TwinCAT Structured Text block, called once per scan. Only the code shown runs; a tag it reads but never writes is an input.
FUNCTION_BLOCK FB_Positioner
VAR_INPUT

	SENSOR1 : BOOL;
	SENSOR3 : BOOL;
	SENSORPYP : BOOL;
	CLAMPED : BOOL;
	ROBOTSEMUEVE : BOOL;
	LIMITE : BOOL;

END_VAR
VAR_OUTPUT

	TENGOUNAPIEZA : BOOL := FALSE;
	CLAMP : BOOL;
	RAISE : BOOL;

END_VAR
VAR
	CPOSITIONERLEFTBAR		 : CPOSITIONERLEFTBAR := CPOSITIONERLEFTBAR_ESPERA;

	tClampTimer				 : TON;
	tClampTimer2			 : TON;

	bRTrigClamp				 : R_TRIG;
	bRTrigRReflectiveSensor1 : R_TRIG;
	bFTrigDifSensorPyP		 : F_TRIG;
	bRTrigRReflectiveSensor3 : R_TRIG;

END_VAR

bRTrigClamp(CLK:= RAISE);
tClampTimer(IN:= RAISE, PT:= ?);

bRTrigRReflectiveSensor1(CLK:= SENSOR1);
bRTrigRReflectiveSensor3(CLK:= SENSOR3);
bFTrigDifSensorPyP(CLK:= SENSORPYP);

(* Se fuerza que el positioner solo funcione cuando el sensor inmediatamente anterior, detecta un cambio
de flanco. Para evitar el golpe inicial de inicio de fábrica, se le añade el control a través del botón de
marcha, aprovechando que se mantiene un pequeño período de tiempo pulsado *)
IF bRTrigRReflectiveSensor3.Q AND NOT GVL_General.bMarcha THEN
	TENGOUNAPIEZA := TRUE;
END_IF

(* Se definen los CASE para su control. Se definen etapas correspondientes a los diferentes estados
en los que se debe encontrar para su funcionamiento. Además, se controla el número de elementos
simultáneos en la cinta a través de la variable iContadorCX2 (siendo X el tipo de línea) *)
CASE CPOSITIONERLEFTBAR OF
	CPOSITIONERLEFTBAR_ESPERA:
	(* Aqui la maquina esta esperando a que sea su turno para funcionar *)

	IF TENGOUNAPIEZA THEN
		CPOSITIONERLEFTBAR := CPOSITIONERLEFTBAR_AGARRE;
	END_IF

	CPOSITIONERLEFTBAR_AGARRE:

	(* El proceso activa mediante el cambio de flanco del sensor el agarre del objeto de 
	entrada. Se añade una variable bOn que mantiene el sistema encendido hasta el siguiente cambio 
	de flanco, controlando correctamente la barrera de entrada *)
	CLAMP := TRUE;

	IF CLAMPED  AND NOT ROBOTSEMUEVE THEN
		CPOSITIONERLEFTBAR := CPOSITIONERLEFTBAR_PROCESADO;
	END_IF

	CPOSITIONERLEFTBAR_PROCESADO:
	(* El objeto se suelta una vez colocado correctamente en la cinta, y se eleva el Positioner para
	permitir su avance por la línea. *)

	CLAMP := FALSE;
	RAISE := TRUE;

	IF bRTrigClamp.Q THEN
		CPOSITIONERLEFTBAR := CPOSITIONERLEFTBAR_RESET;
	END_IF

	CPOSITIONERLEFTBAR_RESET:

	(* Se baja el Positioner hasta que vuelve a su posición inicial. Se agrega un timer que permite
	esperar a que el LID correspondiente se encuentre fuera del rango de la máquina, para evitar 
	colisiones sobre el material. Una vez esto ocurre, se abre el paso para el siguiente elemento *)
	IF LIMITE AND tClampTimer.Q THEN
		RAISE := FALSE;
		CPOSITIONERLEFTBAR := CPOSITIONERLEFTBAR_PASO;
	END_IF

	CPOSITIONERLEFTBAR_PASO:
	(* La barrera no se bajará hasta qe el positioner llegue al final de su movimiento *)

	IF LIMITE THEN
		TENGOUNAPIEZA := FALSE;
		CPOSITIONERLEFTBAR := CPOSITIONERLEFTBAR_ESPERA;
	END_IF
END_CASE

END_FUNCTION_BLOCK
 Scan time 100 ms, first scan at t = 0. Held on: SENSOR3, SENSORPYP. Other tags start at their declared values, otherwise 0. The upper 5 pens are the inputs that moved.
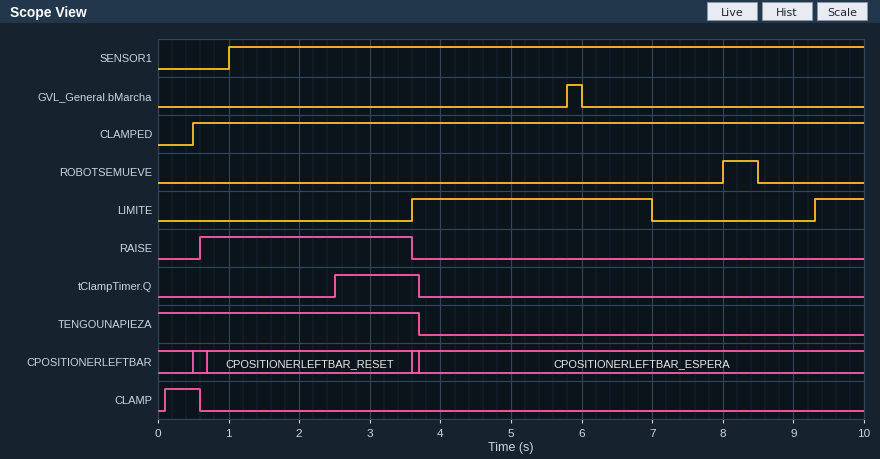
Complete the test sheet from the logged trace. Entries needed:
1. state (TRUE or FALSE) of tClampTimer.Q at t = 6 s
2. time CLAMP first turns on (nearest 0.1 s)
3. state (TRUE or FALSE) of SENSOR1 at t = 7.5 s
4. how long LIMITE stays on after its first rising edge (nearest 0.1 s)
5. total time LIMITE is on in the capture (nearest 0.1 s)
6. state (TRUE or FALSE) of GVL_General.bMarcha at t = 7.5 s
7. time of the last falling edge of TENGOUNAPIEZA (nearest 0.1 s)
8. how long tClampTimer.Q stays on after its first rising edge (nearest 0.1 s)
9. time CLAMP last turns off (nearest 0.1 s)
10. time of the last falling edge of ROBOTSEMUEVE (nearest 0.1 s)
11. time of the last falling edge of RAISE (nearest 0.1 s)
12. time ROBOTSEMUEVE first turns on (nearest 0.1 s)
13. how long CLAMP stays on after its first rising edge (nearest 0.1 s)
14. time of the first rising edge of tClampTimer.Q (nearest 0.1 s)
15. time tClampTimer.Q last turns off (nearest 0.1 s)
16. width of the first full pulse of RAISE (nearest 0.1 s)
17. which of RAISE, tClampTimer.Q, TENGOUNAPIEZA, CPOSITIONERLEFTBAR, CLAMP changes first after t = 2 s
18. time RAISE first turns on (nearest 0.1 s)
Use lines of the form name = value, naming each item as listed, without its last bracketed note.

state (TRUE or FALSE) of tClampTimer.Q at t = 6 s = FALSE
time CLAMP first turns on = 0.1 s
state (TRUE or FALSE) of SENSOR1 at t = 7.5 s = TRUE
how long LIMITE stays on after its first rising edge = 3.4 s
total time LIMITE is on in the capture = 4.1 s
state (TRUE or FALSE) of GVL_General.bMarcha at t = 7.5 s = FALSE
time of the last falling edge of TENGOUNAPIEZA = 3.7 s
how long tClampTimer.Q stays on after its first rising edge = 1.2 s
time CLAMP last turns off = 0.6 s
time of the last falling edge of ROBOTSEMUEVE = 8.5 s
time of the last falling edge of RAISE = 3.6 s
time ROBOTSEMUEVE first turns on = 8.0 s
how long CLAMP stays on after its first rising edge = 0.5 s
time of the first rising edge of tClampTimer.Q = 2.5 s
time tClampTimer.Q last turns off = 3.7 s
width of the first full pulse of RAISE = 3.0 s
which of RAISE, tClampTimer.Q, TENGOUNAPIEZA, CPOSITIONERLEFTBAR, CLAMP changes first after t = 2 s = tClampTimer.Q
time RAISE first turns on = 0.6 s
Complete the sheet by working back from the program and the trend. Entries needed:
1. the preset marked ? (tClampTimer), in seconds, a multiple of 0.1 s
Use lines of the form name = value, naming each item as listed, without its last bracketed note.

the preset marked ? (tClampTimer), in seconds, a multiple of 0.1 s = 1.8 s
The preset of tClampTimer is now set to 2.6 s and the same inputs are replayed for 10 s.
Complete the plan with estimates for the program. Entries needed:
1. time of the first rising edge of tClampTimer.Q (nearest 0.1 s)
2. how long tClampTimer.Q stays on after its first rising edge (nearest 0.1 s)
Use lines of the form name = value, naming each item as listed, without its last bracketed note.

time of the first rising edge of tClampTimer.Q = 3.3 s
how long tClampTimer.Q stays on after its first rising edge = 0.4 s
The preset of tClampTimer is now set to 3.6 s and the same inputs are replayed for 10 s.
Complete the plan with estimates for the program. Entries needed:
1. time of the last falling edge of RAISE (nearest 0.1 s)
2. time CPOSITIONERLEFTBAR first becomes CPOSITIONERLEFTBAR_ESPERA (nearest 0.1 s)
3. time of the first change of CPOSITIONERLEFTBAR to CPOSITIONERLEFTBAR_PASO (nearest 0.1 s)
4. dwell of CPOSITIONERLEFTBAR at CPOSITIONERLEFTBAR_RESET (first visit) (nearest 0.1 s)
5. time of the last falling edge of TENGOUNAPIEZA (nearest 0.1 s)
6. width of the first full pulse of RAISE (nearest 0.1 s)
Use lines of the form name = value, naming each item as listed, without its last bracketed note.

time of the last falling edge of RAISE = 4.3 s
time CPOSITIONERLEFTBAR first becomes CPOSITIONERLEFTBAR_ESPERA = 4.4 s
time of the first change of CPOSITIONERLEFTBAR to CPOSITIONERLEFTBAR_PASO = 4.3 s
dwell of CPOSITIONERLEFTBAR at CPOSITIONERLEFTBAR_RESET (first visit) = 3.6 s
time of the last falling edge of TENGOUNAPIEZA = 4.4 s
width of the first full pulse of RAISE = 3.7 s
